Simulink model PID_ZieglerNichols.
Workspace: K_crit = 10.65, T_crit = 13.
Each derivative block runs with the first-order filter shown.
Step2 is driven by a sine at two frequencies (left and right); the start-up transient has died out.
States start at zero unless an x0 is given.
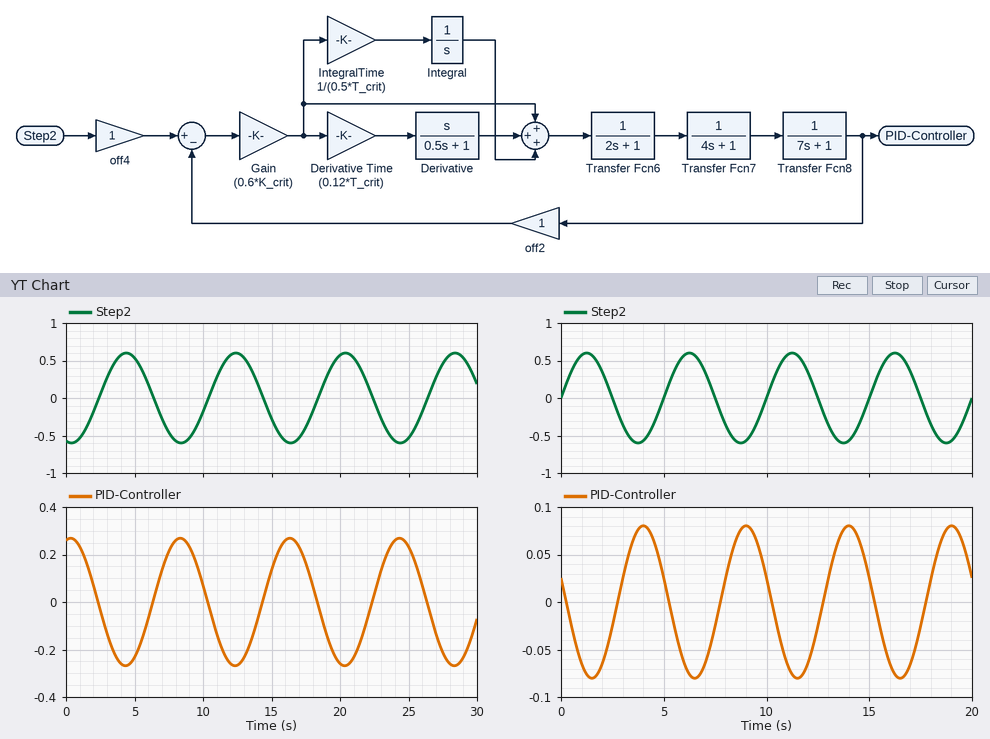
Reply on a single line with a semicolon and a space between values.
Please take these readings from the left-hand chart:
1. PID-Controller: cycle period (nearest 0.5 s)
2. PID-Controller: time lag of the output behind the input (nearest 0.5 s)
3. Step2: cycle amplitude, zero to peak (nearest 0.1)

8.0 s; 4.0 s; 0.6
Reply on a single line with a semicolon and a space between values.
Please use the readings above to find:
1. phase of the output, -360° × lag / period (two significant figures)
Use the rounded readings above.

-180°
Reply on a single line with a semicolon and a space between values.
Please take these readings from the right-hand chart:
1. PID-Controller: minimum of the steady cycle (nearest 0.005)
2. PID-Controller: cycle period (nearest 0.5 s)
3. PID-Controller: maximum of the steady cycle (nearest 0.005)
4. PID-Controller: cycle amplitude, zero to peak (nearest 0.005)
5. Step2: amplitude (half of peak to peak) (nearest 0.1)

-0.080; 5.0 s; 0.080; 0.080; 0.6
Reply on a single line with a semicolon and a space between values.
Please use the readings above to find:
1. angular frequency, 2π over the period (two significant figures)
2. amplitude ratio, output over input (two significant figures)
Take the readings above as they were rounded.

1.3 rad/s; 0.13
